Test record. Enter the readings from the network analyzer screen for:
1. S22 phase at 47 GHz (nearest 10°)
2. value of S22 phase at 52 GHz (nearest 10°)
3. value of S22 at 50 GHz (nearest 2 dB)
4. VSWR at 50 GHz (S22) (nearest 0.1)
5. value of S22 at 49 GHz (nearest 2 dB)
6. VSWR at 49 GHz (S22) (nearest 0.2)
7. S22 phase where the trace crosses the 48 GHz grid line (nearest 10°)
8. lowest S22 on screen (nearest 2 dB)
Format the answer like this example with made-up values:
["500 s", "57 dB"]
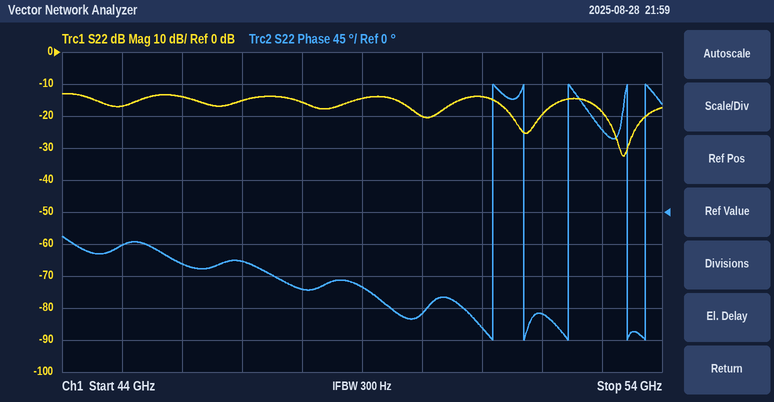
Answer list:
["-70°", "-140°", "-20 dB", "1.2", "-14 dB", "1.4", "-110°", "-32 dB"]
